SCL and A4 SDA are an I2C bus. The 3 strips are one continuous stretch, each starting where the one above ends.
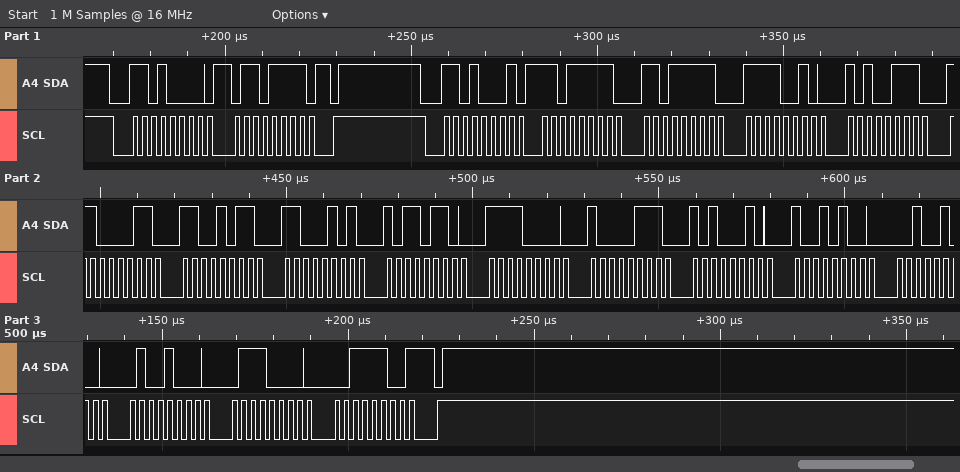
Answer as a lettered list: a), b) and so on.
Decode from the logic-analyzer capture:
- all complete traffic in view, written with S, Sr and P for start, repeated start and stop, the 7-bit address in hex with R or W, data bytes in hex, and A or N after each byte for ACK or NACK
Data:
a) S 68W A 6F A P S 68R A DF A DF A F2 A A7 A C3 A CB A C5 A B6 A F0 A 87 A A2 A 94 A 24 A 48 A 70 A 3C N P
